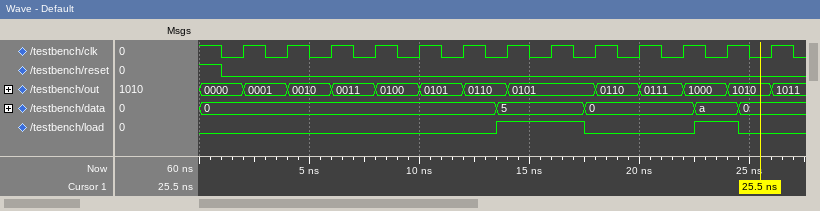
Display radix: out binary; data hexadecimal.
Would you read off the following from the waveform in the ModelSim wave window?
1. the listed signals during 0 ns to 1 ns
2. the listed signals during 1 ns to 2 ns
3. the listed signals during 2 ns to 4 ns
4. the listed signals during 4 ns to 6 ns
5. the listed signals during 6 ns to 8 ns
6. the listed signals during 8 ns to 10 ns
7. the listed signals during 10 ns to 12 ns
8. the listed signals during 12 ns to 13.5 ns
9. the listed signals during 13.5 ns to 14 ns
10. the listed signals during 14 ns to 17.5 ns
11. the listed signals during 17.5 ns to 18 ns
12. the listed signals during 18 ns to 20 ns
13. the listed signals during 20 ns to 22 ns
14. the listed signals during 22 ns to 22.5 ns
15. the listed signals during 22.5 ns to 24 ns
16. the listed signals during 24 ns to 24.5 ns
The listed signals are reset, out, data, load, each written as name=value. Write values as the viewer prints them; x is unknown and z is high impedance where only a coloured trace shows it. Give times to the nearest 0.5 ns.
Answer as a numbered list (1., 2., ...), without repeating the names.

1. reset=1, out=0000, data=0, load=0
2. reset=0, out=0000, data=0, load=0
3. reset=0, out=0001, data=0, load=0
4. reset=0, out=0010, data=0, load=0
5. reset=0, out=0011, data=0, load=0
6. reset=0, out=0100, data=0, load=0
7. reset=0, out=0101, data=0, load=0
8. reset=0, out=0110, data=0, load=0
9. reset=0, out=0110, data=5, load=1
10. reset=0, out=0101, data=5, load=1
11. reset=0, out=0101, data=0, load=0
12. reset=0, out=0110, data=0, load=0
13. reset=0, out=0111, data=0, load=0
14. reset=0, out=1000, data=0, load=0
15. reset=0, out=1000, data=a, load=1
16. reset=0, out=1010, data=a, load=1
